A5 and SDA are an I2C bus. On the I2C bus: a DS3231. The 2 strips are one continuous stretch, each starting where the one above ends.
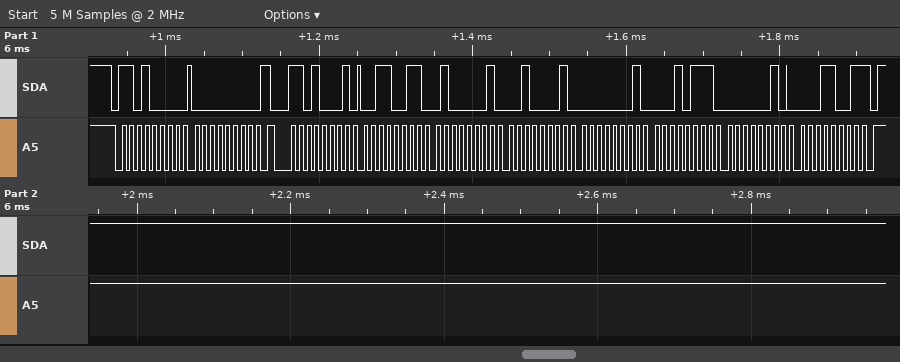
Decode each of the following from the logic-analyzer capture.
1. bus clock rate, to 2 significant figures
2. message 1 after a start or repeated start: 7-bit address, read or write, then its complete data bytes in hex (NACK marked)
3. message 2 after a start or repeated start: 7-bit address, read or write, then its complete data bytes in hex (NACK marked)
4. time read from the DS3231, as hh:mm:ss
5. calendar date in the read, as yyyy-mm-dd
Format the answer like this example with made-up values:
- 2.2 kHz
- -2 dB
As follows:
- 100 kHz
- 0x68 write: 00
- 0x68 read: 33 41 21 01 17 02 19 NACK
- 21:41:33
- 2019-02-17
